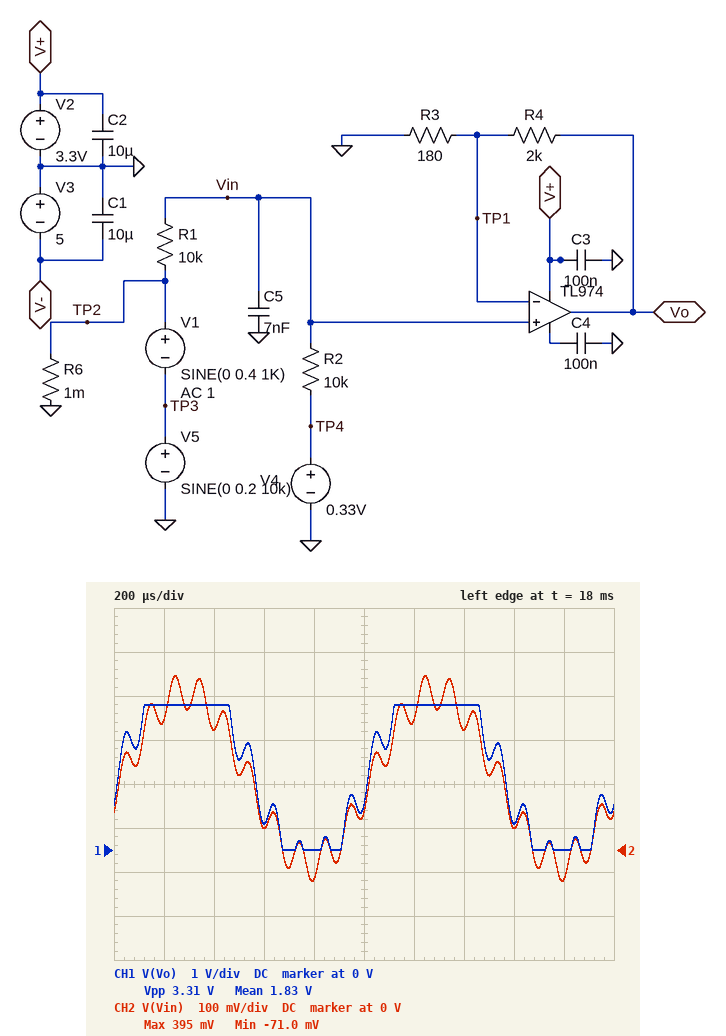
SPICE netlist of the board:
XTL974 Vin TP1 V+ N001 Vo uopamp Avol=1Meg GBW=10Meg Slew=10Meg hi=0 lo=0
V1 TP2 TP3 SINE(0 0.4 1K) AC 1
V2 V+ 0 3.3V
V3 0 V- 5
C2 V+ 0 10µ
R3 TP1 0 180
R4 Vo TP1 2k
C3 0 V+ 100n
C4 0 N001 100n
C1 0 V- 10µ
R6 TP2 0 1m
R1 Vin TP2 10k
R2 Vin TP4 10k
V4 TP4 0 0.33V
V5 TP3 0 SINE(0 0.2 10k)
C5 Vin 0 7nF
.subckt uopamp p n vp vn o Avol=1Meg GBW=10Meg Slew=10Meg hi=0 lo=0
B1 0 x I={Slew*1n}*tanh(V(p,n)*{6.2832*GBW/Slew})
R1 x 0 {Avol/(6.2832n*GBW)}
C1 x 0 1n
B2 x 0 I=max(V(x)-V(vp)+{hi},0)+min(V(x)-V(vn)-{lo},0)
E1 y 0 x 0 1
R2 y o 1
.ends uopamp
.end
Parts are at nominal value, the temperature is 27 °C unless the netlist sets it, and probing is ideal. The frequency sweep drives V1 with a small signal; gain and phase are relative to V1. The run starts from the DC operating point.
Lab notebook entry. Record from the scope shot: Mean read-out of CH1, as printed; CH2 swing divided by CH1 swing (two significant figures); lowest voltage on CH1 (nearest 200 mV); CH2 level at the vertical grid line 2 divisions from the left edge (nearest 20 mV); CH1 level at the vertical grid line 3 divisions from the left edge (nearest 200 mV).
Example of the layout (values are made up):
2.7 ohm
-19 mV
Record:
1.83 V
0.14
0 V
280 mV
600 mV
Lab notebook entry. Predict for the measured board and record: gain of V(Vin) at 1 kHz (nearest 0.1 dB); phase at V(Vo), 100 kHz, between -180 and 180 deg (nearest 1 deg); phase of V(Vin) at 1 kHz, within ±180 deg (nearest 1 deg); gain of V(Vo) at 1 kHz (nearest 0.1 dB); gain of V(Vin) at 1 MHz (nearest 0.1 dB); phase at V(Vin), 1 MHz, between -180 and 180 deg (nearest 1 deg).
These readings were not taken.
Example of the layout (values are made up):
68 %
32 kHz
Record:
-6.2 dB
-94 deg
-12 deg
15.4 dB
-52.9 dB
-90 deg
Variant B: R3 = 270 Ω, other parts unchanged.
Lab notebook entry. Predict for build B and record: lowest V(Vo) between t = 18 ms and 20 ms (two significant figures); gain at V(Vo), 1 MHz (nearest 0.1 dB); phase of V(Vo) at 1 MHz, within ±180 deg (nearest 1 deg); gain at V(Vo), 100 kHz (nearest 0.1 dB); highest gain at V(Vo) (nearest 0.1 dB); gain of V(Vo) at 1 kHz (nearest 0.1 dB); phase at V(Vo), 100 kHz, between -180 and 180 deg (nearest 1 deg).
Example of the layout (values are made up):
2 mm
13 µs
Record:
-4.2 mV
-36.7 dB
-130 deg
-14.4 dB
12.5 dB
12.3 dB
-92 deg
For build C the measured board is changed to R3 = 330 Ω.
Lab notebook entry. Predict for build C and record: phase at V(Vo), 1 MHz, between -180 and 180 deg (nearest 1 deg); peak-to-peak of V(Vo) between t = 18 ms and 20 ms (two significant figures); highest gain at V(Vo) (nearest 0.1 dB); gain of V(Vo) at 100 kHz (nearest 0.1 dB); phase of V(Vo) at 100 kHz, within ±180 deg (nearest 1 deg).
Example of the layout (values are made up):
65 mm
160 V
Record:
-125 deg
2.8 V
11.0 dB
-15.9 dB
-91 deg
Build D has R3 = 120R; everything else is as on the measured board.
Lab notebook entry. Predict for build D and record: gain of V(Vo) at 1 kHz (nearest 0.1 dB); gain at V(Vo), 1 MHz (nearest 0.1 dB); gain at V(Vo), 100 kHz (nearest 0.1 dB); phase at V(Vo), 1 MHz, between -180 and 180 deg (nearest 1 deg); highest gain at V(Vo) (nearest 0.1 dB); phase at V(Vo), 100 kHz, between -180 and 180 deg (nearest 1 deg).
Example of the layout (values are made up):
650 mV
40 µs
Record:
18.7 dB
-34.1 dB
-8.1 dB
-150 deg
18.9 dB
-97 deg
